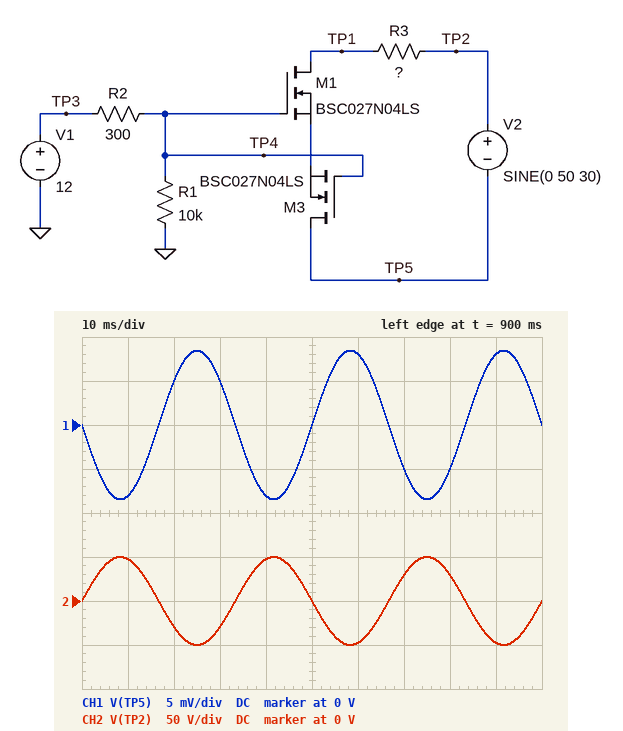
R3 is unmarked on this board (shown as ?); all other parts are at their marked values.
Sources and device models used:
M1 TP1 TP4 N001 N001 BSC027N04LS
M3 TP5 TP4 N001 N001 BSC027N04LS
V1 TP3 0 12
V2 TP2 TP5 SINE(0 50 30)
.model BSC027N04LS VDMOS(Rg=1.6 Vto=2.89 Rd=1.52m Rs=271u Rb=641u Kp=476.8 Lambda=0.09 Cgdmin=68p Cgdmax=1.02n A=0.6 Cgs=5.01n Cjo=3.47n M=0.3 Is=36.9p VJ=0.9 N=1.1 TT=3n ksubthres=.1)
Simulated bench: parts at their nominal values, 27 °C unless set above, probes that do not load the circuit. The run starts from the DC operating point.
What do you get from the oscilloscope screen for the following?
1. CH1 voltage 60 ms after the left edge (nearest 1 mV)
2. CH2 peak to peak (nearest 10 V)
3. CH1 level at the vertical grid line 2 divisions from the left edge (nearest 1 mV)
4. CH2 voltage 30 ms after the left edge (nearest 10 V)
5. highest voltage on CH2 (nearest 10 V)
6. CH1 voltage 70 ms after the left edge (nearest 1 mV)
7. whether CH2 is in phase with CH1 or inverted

8 mV
100 V
5 mV
-30 V
50 V
-5 mV
inverted
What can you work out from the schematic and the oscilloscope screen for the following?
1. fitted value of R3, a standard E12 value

12 Ω
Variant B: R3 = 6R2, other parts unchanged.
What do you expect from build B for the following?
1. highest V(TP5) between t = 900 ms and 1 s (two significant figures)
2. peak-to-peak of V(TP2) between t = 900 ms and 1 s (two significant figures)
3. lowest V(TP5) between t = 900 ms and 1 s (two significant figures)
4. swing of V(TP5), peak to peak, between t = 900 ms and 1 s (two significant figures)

16 mV
100 V
-16 mV
33 mV
